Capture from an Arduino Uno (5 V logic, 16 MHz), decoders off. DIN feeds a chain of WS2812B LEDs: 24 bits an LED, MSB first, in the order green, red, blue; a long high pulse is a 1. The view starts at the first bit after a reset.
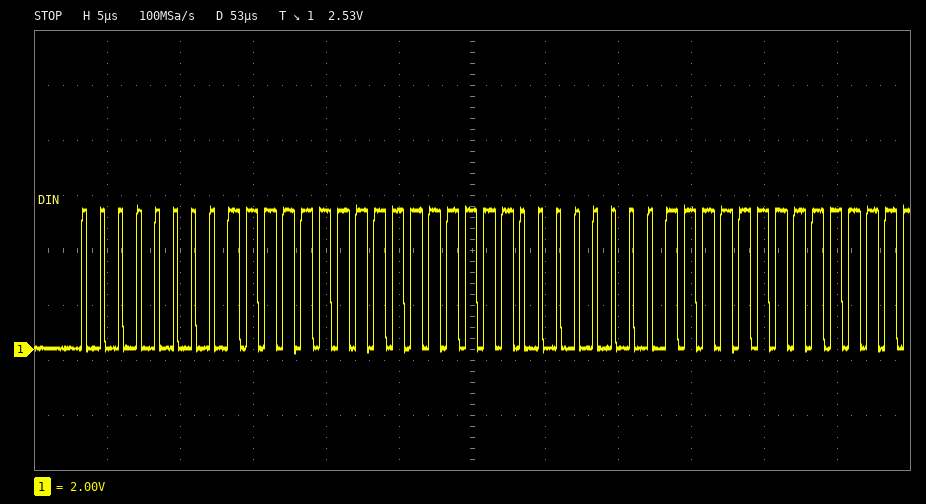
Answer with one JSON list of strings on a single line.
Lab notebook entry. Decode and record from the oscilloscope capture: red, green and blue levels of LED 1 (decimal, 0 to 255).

["255, 0, 255"]
